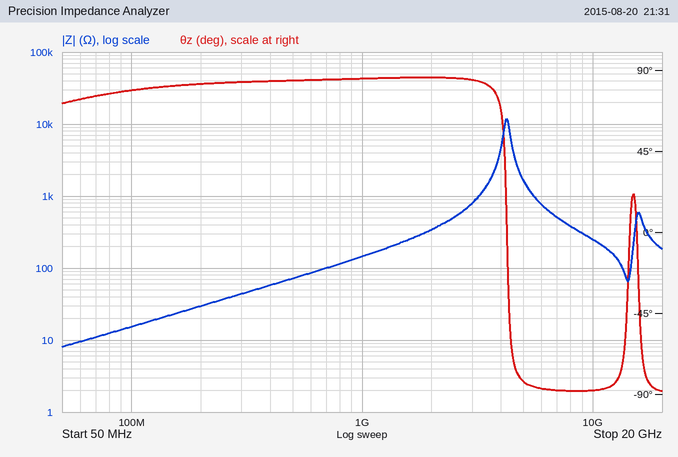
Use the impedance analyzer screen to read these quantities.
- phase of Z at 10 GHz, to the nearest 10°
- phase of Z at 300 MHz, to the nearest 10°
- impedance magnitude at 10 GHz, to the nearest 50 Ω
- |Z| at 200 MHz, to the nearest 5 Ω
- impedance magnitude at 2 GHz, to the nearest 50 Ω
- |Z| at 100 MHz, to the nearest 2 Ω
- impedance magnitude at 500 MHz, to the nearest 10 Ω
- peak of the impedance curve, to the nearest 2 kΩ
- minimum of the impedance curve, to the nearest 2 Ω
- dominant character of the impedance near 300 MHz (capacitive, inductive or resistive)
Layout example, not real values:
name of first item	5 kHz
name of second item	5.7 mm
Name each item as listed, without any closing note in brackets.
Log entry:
phase of Z at 10 GHz, to the nearest 10°	-90°
phase of Z at 300 MHz, to the nearest 10°	80°
impedance magnitude at 10 GHz, to the nearest 50 Ω	250 Ω
|Z| at 200 MHz, to the nearest 5 Ω	30 Ω
impedance magnitude at 2 GHz, to the nearest 50 Ω	350 Ω
|Z| at 100 MHz, to the nearest 2 Ω	16 Ω
impedance magnitude at 500 MHz, to the nearest 10 Ω	70 Ω
peak of the impedance curve, to the nearest 2 kΩ	12 kΩ
minimum of the impedance curve, to the nearest 2 Ω	8 Ω
dominant character of the impedance near 300 MHz	inductive
